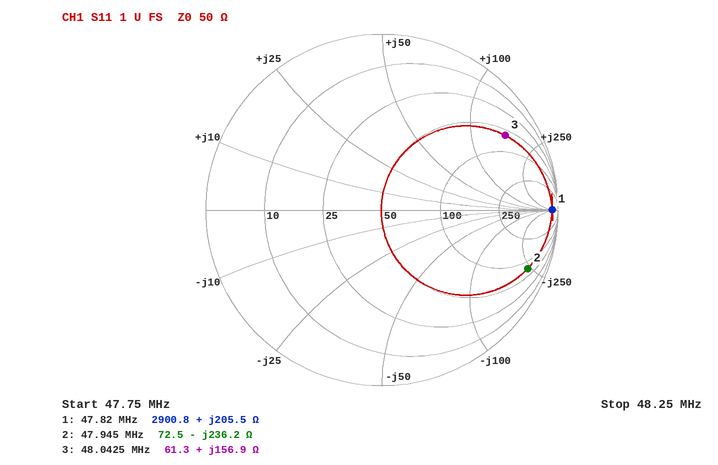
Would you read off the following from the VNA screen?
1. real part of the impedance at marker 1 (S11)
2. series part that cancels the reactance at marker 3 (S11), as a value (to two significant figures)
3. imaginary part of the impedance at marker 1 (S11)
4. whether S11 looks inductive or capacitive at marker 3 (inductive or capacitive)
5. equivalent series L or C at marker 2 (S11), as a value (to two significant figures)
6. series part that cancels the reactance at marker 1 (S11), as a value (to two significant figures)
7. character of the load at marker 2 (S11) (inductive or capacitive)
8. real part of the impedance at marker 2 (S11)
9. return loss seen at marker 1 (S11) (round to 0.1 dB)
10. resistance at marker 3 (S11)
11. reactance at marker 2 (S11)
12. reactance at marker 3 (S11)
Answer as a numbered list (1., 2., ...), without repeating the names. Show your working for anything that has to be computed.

1. 2900.8 Ω
2. C = 1/(2π × 48.0425 MHz × 156.9 Ω) ≈ 21 pF
3. +205.5 Ω
4. inductive
5. C = 1/(2π × 47.945 MHz × 236.2 Ω) ≈ 14 pF
6. C = 1/(2π × 47.82 MHz × 205.5 Ω) ≈ 16 pF
7. capacitive
8. 72.5 Ω
9. 0.3 dB
10. 61.3 Ω
11. -236.2 Ω
12. +156.9 Ω
